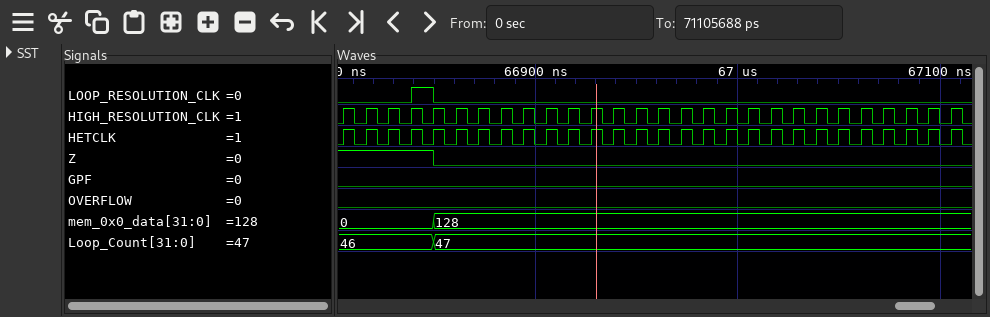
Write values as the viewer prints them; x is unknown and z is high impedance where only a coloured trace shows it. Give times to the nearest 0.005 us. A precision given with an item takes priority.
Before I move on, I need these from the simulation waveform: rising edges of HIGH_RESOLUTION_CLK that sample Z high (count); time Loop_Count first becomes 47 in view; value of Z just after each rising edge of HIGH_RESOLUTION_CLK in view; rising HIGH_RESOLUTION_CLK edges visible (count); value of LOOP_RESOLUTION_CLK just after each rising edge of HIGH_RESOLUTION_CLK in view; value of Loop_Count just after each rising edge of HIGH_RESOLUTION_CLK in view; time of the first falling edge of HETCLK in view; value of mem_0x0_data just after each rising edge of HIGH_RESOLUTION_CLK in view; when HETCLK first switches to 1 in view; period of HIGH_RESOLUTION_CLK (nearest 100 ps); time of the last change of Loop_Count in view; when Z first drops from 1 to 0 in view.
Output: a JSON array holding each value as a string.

["5", "66.85 us", "1 1 1 1 0 0 0 0 0 0 0 0 0 0 0 0 0 0 0 0 0 0 0 0 0 0 0 0", "28", "0 0 0 1 0 0 0 0 0 0 0 0 0 0 0 0 0 0 0 0 0 0 0 0 0 0 0 0", "46, 46, 46, 46, 47, 47, 47, 47, 47, 47, 47, 47, 47, 47, 47, 47, 47, 47, 47, 47, 47, 47, 47, 47, 47, 47, 47, 47", "66.81 us", "0, 0, 0, 0, 128, 128, 128, 128, 128, 128, 128, 128, 128, 128, 128, 128, 128, 128, 128, 128, 128, 128, 128, 128, 128, 128, 128, 128", "66.805 us", "11100 ps", "66.85 us", "66.85 us"]
